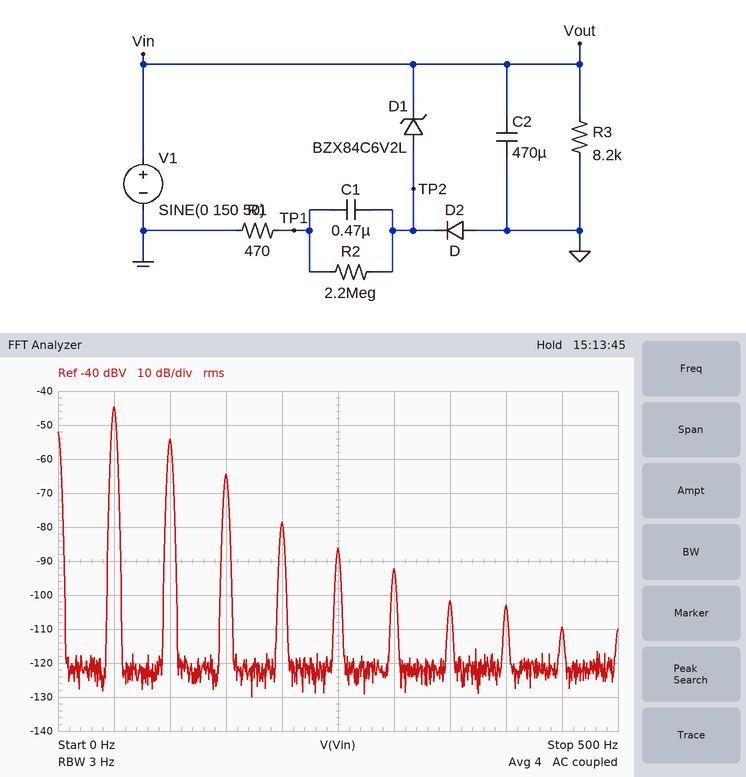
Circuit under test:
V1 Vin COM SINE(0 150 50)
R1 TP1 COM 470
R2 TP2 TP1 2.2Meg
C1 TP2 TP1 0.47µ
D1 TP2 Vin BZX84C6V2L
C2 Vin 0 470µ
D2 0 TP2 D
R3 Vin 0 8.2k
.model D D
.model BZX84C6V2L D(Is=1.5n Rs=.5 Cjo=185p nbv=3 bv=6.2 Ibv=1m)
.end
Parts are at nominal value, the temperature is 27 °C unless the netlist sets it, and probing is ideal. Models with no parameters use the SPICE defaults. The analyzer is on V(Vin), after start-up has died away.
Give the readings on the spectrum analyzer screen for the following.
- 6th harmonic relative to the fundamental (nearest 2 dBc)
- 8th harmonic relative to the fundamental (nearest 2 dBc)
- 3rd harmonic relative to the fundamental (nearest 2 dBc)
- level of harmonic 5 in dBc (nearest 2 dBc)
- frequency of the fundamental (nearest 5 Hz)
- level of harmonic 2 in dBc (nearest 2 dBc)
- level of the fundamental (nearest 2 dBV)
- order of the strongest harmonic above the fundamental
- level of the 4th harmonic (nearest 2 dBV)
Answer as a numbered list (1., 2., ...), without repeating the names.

1. -48 dBc
2. -58 dBc
3. -20 dBc
4. -42 dBc
5. 50 Hz
6. -10 dBc
7. -44 dBV
8. 2
9. -78 dBV
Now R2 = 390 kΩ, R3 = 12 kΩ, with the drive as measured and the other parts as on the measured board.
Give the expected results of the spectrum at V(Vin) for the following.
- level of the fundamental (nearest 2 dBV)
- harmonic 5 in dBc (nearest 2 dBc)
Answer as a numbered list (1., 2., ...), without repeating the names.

1. -48 dBV
2. -44 dBc
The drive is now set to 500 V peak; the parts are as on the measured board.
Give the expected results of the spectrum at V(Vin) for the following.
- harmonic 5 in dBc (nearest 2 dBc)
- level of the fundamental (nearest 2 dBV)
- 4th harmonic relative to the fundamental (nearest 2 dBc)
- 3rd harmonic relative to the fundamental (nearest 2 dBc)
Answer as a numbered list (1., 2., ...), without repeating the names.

1. -40 dBc
2. -44 dBV
3. -28 dBc
4. -18 dBc
